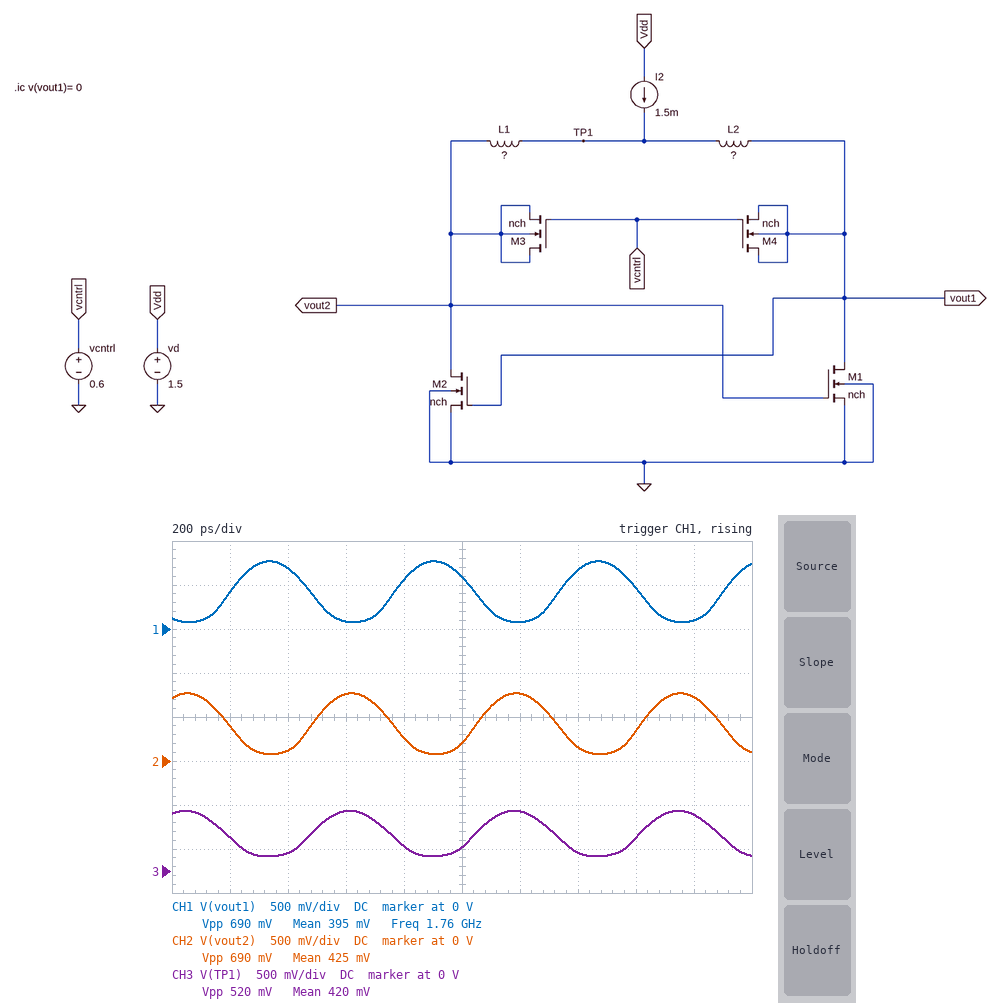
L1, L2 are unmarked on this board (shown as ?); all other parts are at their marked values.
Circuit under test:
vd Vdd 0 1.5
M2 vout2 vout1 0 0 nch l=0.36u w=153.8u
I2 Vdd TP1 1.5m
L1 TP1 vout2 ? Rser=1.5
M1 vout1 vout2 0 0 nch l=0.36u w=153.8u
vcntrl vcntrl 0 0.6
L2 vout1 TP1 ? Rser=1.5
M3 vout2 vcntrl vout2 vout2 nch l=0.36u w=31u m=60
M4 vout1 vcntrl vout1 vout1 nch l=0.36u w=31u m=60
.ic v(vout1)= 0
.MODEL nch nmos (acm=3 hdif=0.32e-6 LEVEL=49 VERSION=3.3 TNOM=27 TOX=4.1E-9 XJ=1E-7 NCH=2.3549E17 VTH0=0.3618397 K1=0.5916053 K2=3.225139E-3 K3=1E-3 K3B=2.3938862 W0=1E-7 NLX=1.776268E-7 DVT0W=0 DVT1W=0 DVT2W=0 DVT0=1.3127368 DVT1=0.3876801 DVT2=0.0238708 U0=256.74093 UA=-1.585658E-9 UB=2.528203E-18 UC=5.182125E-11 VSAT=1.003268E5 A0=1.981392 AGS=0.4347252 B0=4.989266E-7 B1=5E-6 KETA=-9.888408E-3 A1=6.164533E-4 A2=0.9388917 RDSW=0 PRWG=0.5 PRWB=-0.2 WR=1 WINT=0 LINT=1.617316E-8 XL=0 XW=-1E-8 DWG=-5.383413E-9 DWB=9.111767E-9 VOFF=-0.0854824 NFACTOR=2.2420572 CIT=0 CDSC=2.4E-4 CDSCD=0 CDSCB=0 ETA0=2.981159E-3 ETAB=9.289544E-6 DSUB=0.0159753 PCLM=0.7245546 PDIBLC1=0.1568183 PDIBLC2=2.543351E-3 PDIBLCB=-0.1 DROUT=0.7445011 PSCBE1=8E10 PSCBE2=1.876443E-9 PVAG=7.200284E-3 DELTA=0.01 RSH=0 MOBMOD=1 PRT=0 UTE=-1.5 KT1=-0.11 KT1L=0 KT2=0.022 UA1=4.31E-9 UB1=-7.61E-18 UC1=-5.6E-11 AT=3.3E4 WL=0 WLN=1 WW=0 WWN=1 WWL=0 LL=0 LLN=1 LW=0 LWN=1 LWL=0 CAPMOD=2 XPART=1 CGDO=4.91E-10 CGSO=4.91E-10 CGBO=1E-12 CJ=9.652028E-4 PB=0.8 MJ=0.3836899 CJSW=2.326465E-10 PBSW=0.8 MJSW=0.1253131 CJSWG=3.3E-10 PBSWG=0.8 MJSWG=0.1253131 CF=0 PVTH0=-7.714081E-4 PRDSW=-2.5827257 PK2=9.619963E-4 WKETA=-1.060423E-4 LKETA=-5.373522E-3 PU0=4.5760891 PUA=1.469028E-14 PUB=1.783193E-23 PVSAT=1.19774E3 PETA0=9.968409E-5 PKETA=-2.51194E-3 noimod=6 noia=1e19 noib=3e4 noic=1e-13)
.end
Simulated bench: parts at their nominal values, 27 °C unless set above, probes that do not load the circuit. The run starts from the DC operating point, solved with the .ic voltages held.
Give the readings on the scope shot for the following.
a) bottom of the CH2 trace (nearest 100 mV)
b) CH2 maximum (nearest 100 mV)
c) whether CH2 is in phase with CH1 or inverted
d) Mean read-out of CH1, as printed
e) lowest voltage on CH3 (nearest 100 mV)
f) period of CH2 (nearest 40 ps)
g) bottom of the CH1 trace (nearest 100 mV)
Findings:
100 mV
800 mV
inverted
395 mV
200 mV
560 ps
100 mV
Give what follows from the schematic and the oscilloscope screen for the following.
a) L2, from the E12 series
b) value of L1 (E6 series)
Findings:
3.3 nH
470 pH
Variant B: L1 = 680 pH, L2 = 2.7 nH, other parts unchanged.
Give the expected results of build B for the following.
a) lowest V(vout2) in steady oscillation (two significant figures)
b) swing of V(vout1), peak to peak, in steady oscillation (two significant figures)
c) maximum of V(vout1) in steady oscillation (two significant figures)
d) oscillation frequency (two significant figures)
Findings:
100 mV
650 mV
750 mV
1.9 GHz
